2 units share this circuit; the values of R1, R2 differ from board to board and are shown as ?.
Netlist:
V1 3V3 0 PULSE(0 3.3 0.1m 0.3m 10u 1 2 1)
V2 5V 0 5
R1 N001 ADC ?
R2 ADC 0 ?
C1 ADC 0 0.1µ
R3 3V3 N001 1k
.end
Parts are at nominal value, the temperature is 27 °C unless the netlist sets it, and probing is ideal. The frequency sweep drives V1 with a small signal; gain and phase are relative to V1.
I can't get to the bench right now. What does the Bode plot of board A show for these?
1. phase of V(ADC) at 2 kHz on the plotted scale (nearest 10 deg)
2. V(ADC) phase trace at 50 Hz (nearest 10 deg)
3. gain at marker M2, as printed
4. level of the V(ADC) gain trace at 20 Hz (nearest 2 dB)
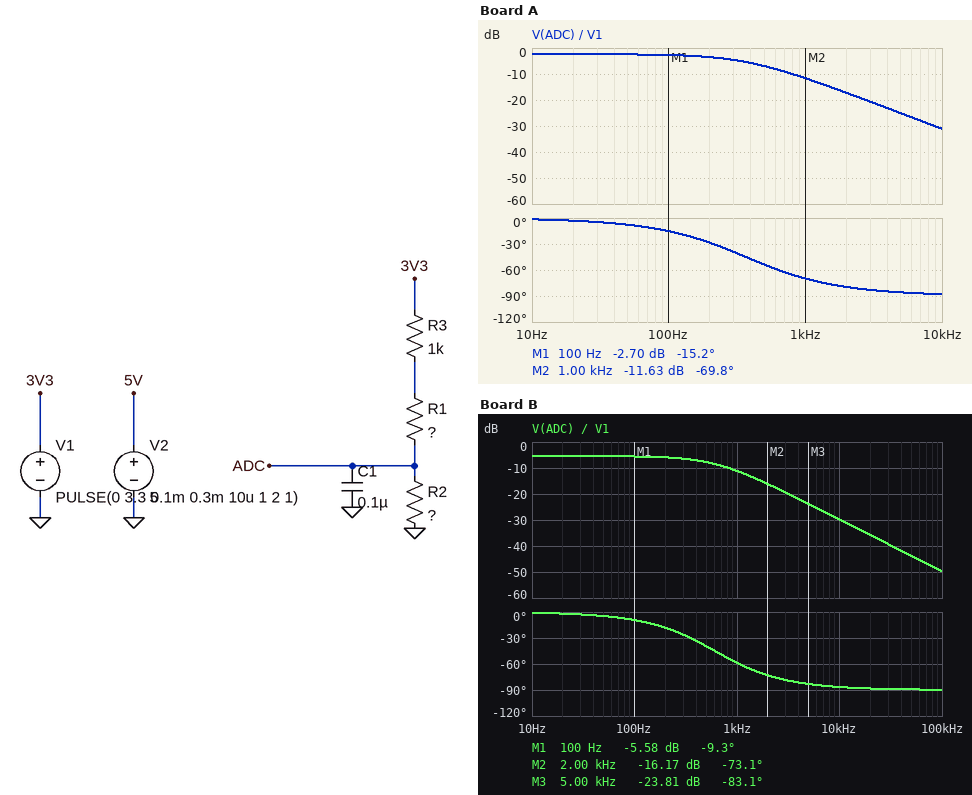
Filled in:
-80 deg
-10 deg
-11.63 dB
-2 dB
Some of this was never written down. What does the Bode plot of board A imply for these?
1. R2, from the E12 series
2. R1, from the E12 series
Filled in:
18 kΩ
4.7 kΩ
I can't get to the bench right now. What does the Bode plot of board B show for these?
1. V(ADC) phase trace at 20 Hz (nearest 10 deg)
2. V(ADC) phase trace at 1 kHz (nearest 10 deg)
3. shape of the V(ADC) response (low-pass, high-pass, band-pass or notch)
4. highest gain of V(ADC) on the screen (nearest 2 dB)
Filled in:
0 deg
-60 deg
low-pass
-6 dB
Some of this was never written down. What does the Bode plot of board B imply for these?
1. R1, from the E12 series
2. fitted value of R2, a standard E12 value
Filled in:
3.9 kΩ
5.6 kΩ
